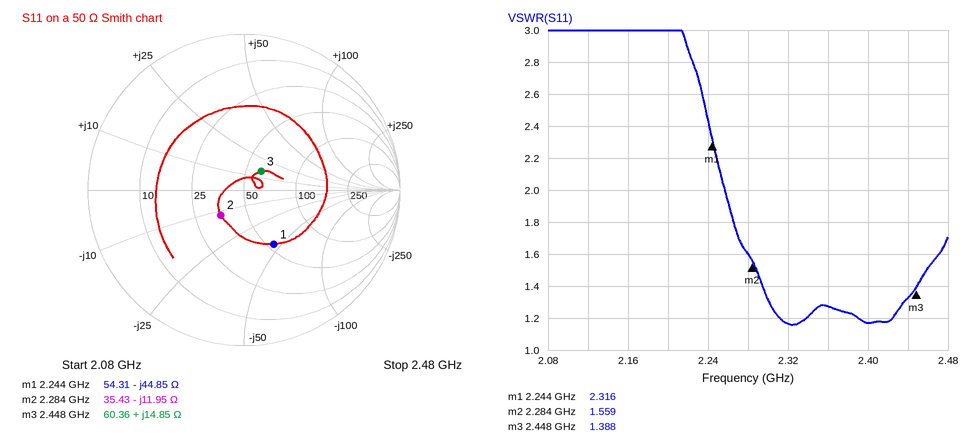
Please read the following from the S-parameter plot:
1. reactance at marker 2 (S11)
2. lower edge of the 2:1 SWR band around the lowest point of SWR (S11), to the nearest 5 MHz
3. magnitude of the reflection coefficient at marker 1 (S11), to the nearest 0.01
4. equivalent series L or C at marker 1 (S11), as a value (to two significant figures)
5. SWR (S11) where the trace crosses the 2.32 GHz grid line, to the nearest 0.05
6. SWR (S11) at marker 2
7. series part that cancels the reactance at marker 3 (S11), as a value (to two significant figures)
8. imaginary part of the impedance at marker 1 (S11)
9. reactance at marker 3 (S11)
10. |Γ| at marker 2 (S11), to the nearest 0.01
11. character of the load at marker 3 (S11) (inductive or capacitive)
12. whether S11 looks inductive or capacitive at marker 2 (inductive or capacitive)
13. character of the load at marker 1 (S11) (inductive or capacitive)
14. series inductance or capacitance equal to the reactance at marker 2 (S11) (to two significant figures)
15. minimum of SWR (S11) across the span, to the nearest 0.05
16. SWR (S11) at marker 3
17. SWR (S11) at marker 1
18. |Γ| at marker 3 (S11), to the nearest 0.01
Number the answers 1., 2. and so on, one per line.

1. -11.95 Ω
2. 2.255 GHz
3. 0.40
4. 1.6 pF
5. 1.15
6. 1.559
7. 4.4 pF
8. -44.85 Ω
9. +14.85 Ω
10. 0.22
11. inductive
12. capacitive
13. capacitive
14. 5.8 pF
15. 1.15
16. 1.388
17. 2.316
18. 0.16
